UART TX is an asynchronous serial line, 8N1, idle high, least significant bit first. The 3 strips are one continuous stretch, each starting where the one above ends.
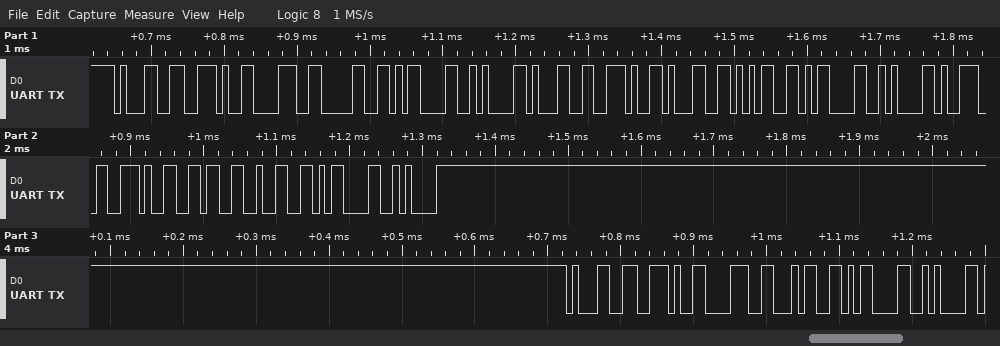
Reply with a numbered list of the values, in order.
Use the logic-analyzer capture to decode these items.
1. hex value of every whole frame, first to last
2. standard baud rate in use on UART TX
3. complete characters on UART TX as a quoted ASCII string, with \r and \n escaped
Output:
1. 31 2E 38 30 0D 0A 31 2E 31 35 0D 0A 39 2E 36 32 0D 0A 31 2E 38 34 0D 0A
2. 115200 baud
3. "1.80\r\n1.15\r\n9.62\r\n1.84\r\n"
